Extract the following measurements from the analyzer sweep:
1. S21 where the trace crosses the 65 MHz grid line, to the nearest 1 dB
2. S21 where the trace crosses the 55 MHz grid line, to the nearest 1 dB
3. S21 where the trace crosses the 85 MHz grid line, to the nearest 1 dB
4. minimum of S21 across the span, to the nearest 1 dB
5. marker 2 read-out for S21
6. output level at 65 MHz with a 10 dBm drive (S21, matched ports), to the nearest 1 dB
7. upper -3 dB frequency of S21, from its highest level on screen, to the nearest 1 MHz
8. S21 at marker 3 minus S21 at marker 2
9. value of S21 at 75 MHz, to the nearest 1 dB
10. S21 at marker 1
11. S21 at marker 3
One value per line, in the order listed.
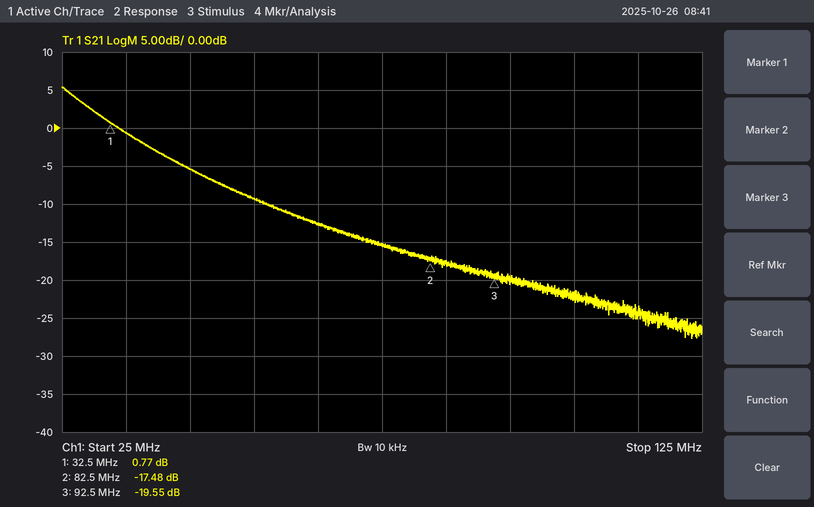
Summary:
-13 dB
-9 dB
-18 dB
-28 dB
-17.48 dB
-3 dBm
30 MHz
-2.07 dB
-15 dB
0.77 dB
-19.55 dB
